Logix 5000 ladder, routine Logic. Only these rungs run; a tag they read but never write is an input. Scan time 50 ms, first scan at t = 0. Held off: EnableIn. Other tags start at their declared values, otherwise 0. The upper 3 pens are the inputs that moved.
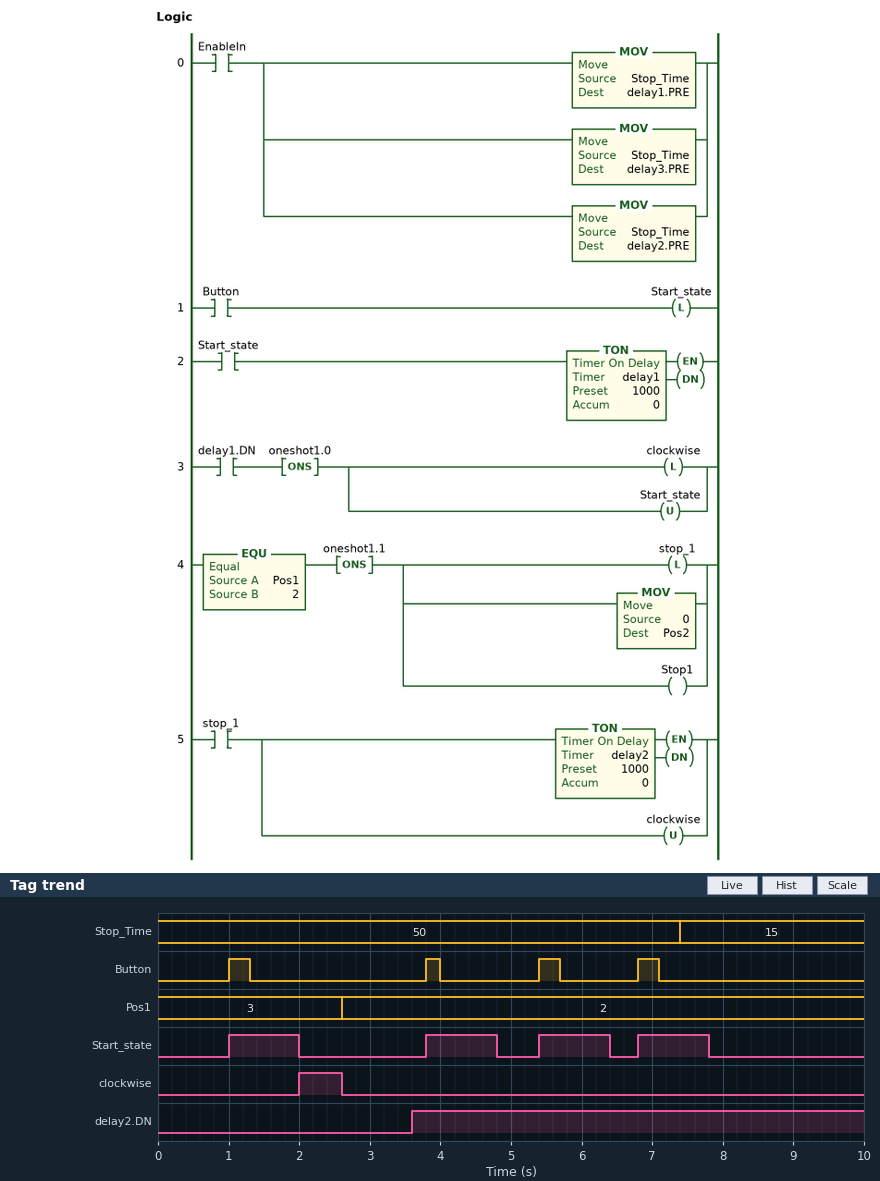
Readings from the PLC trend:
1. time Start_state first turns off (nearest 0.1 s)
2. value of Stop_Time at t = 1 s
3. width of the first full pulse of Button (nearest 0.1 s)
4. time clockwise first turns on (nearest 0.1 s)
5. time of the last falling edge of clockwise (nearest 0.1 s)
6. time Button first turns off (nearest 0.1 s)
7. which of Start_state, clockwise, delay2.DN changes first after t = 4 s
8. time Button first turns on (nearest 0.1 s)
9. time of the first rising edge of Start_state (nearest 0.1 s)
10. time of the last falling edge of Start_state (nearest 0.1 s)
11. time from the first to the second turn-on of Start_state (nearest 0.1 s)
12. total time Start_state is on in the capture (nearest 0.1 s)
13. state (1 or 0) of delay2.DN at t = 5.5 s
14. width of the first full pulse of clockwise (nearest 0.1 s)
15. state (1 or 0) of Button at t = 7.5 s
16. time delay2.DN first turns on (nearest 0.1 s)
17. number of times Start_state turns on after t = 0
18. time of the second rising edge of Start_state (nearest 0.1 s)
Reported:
2.0 s
50
0.3 s
2.0 s
2.6 s
1.3 s
Start_state
1.0 s
1.0 s
7.8 s
2.8 s
4.0 s
1
0.6 s
0
3.6 s
4
3.8 s
